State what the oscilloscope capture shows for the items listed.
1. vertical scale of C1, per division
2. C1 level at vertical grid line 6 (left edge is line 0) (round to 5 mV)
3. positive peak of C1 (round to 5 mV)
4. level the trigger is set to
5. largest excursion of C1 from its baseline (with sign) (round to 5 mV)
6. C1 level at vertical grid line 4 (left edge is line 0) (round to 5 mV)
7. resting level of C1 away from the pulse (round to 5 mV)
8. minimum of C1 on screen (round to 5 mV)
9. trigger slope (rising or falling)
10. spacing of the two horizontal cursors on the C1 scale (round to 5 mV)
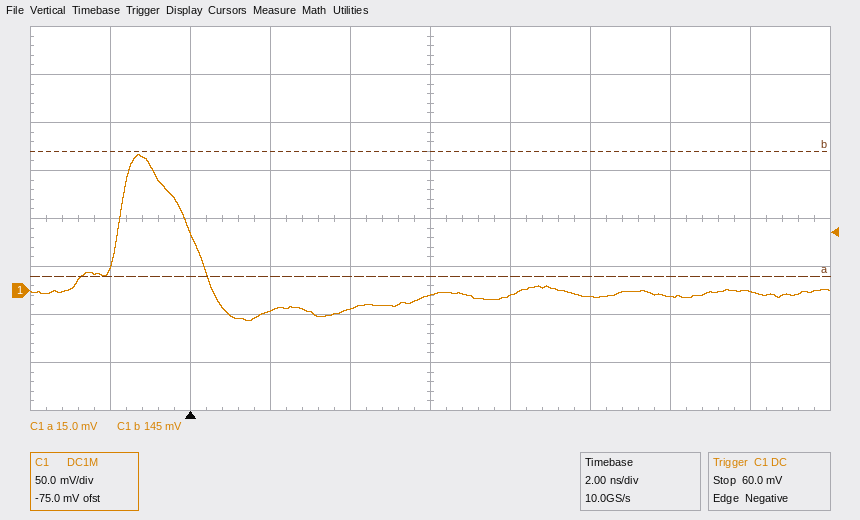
50 mV
-5 mV
140 mV
60.0 mV
+145 mV
-20 mV
-5 mV
-30 mV
falling
130 mV
